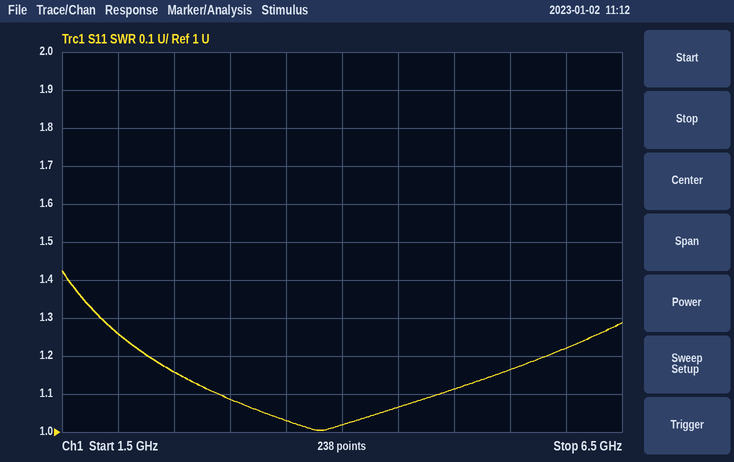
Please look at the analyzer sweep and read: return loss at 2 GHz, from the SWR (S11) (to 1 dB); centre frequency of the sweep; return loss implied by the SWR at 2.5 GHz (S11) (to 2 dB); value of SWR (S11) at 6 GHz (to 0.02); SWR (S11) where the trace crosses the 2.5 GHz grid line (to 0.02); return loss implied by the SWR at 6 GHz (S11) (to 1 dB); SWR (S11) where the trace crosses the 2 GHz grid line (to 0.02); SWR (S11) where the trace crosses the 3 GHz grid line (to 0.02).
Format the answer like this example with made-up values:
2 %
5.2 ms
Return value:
19 dB
4 GHz
22 dB
1.22
1.16
20 dB
1.26
1.08
